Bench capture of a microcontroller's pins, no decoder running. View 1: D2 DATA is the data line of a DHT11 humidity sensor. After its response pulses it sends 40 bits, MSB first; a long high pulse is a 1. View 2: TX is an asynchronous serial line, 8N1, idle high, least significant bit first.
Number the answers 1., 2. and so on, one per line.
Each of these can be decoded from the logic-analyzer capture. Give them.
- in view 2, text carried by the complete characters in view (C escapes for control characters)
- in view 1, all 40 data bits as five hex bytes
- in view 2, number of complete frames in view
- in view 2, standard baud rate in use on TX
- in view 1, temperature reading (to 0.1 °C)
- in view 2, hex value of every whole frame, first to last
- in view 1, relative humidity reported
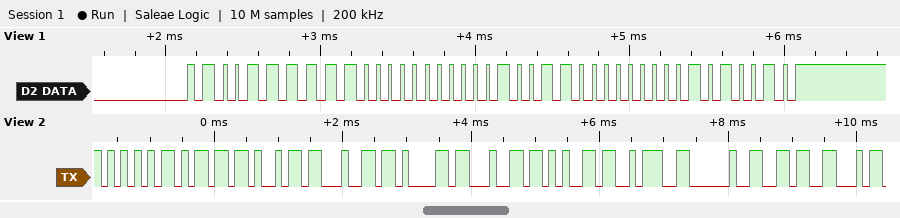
1. "Umidade: 6"
2. 3F 00 13 00 52
3. 10
4. 9600 baud
5. 19.0 °C
6. 55 6D 69 64 61 64 65 3A 20 36
7. 63 %
